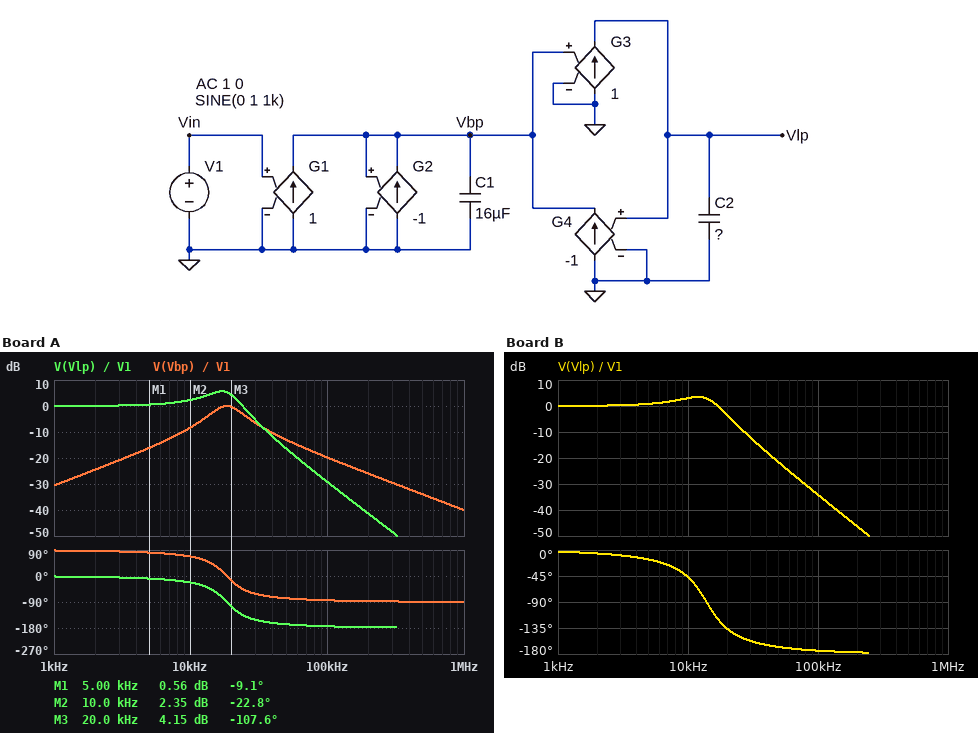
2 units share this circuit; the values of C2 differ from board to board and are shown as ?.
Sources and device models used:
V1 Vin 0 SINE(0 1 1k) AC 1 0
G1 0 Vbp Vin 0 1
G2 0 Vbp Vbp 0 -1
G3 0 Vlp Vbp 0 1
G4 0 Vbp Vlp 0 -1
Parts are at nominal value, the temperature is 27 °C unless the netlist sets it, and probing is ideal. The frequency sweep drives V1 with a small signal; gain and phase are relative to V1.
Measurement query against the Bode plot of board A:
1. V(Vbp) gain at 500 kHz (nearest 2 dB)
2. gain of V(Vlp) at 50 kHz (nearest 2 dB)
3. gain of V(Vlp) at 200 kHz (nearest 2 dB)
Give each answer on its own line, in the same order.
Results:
-34 dB
-16 dB
-42 dB
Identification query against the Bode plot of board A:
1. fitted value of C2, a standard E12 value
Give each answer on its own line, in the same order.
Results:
4.7 µF
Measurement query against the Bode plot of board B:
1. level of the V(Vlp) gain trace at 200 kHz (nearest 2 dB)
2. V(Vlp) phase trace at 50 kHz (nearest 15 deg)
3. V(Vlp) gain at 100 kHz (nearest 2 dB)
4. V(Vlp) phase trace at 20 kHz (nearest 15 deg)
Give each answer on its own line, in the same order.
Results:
-46 dB
-165 deg
-34 dB
-135 deg
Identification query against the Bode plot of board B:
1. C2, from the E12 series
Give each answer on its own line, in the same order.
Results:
8.2 µF
